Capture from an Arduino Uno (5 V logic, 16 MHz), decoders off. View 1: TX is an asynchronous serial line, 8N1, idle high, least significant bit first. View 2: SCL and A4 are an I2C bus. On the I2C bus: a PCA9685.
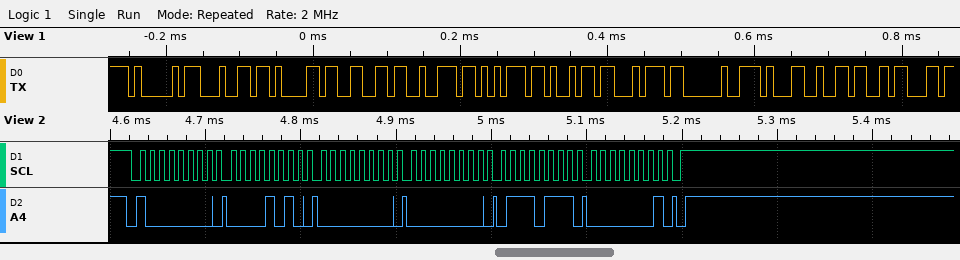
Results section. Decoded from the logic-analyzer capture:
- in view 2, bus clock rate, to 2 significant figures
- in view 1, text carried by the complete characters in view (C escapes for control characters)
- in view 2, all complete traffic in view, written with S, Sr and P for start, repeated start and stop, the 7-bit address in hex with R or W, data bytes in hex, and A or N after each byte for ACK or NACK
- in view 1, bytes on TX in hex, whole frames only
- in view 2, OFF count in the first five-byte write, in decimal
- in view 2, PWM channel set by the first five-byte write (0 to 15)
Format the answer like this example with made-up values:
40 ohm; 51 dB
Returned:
100 kHz; "Adafruit 16c"; S 40W A 0A A 00 A 00 A 77 A 01 A P; 41 64 61 66 72 75 69 74 20 31 36 63; 375; 1
